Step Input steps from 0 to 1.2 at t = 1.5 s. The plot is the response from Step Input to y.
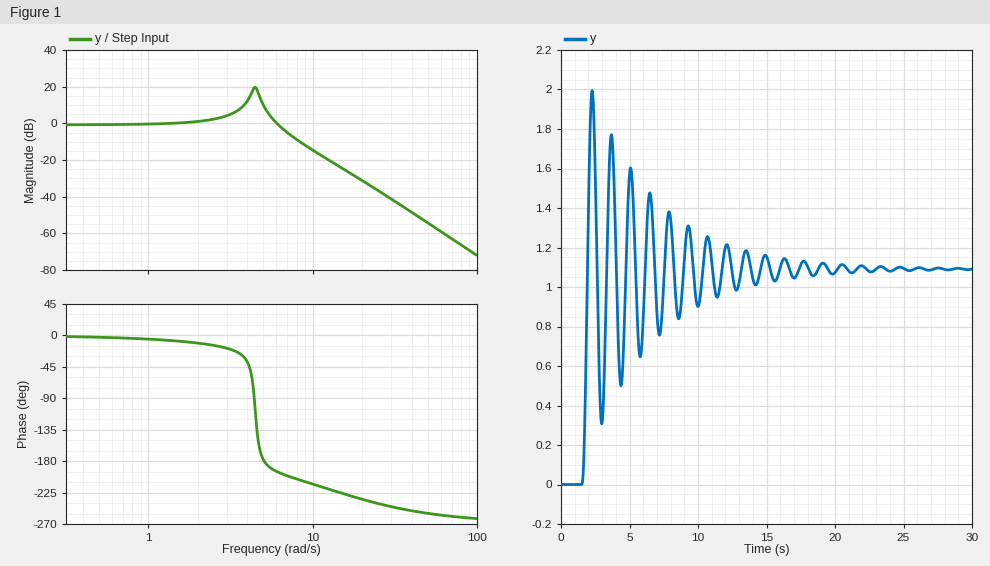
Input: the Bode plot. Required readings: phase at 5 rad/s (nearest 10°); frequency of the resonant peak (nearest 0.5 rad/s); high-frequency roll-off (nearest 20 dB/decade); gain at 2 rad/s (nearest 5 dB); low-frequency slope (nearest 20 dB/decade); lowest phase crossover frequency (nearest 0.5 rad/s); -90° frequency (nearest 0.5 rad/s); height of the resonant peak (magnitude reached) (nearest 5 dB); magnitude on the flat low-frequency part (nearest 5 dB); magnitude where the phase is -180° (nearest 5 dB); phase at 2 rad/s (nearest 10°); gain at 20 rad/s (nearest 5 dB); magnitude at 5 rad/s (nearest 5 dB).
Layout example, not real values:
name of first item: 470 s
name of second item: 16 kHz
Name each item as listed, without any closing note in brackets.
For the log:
phase at 5 rad/s: -180°
frequency of the resonant peak: 4.5 rad/s
high-frequency roll-off: -60 dB/decade
gain at 2 rad/s: 0 dB
low-frequency slope: 0 dB/decade
lowest phase crossover frequency: 5.0 rad/s
-90° frequency: 4.5 rad/s
height of the resonant peak (magnitude reached): 20 dB
magnitude on the flat low-frequency part: 0 dB
magnitude where the phase is -180°: 10 dB
phase at 2 rad/s: -10°
gain at 20 rad/s: -30 dB
magnitude at 5 rad/s: 10 dB
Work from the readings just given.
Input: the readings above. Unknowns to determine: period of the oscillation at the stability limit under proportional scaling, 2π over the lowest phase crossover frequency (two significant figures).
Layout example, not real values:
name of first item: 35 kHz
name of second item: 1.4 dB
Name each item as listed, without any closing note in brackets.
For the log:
period of the oscillation at the stability limit under proportional scaling, 2π over the lowest phase crossover frequency: 1.3 s
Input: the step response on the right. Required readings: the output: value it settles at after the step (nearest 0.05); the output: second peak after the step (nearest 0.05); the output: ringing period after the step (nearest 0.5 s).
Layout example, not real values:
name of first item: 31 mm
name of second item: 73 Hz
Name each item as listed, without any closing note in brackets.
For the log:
the output: value it settles at after the step: 1.10
the output: second peak after the step: 1.75
the output: ringing period after the step: 1.5 s
